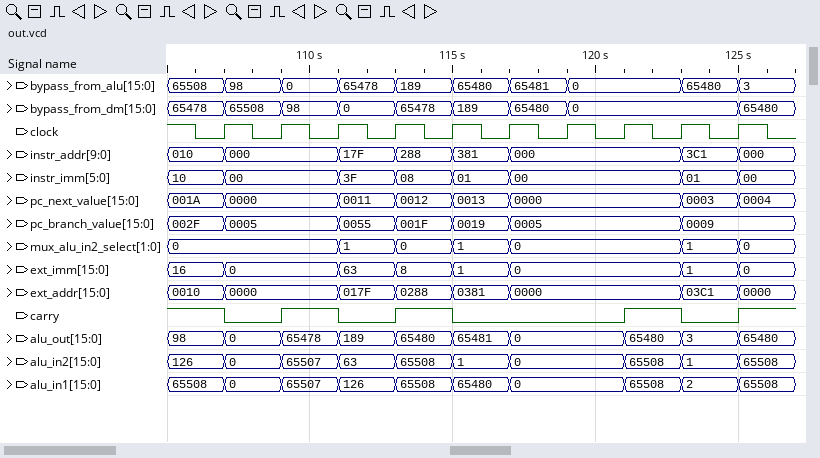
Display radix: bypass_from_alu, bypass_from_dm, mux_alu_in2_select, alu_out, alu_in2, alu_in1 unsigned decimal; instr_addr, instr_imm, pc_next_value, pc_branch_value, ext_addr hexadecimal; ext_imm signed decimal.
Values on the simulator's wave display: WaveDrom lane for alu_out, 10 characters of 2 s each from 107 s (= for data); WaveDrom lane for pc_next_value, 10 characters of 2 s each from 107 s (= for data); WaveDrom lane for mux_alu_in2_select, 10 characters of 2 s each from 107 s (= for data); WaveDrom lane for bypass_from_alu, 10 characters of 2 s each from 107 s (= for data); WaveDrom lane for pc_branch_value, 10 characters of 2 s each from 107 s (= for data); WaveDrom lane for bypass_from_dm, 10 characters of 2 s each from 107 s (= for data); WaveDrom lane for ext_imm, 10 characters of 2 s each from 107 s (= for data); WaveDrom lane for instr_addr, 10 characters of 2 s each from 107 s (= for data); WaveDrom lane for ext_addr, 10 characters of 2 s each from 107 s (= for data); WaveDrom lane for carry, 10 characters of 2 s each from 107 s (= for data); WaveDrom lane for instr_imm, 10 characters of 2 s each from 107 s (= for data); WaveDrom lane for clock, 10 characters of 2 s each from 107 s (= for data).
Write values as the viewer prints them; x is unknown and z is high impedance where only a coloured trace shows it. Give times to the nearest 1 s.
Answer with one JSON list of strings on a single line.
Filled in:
["{name: 'alu_out', wave: '======.===', data: '0 65478 189 65480 65481 0 65480 3 65480'}", "{name: 'pc_next_value', wave: '=.====..==', data: '0000 0011 0012 0013 0000 0003 0004'}", "{name: 'mux_alu_in2_select', wave: '=.====..==', data: '0 1 0 1 0 1 0'}", "{name: 'bypass_from_alu', wave: '=======.==', data: '98 0 65478 189 65480 65481 0 65480 3'}", "{name: 'pc_branch_value', wave: '=.====..=.', data: '0005 0055 001F 0019 0005 0009'}", "{name: 'bypass_from_dm', wave: '=======..=', data: '65508 98 0 65478 189 65480 0 65480'}", "{name: 'ext_imm', wave: '=.====..==', data: '0 63 8 1 0 1 0'}", "{name: 'instr_addr', wave: '=.====..==', data: '000 17F 288 381 000 3C1 000'}", "{name: 'ext_addr', wave: '=.====..==', data: '0000 017F 0288 0381 0000 03C1 0000'}", "{name: 'carry', wave: '01010..101'}", "{name: 'instr_imm', wave: '=.====..==', data: '00 3F 08 01 00 01 00'}", "{name: 'clock', wave: 'p.........'}"]
